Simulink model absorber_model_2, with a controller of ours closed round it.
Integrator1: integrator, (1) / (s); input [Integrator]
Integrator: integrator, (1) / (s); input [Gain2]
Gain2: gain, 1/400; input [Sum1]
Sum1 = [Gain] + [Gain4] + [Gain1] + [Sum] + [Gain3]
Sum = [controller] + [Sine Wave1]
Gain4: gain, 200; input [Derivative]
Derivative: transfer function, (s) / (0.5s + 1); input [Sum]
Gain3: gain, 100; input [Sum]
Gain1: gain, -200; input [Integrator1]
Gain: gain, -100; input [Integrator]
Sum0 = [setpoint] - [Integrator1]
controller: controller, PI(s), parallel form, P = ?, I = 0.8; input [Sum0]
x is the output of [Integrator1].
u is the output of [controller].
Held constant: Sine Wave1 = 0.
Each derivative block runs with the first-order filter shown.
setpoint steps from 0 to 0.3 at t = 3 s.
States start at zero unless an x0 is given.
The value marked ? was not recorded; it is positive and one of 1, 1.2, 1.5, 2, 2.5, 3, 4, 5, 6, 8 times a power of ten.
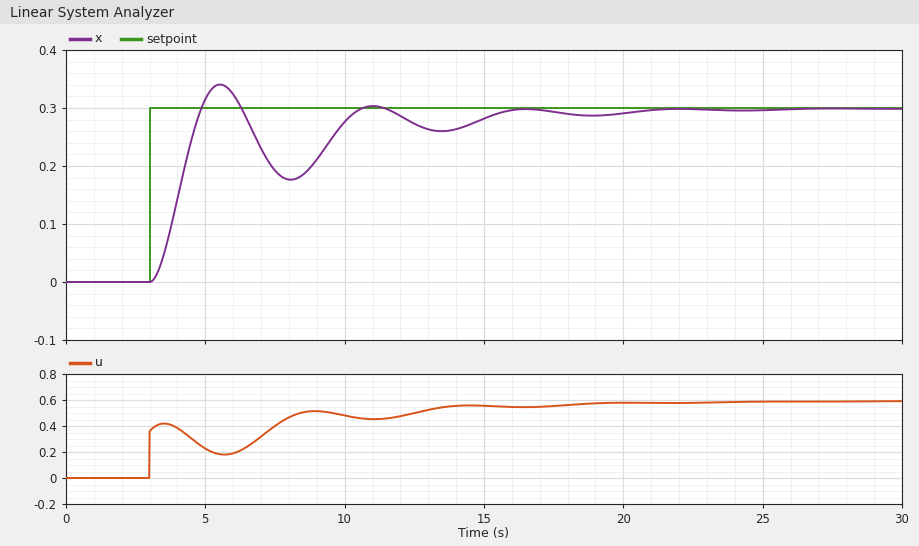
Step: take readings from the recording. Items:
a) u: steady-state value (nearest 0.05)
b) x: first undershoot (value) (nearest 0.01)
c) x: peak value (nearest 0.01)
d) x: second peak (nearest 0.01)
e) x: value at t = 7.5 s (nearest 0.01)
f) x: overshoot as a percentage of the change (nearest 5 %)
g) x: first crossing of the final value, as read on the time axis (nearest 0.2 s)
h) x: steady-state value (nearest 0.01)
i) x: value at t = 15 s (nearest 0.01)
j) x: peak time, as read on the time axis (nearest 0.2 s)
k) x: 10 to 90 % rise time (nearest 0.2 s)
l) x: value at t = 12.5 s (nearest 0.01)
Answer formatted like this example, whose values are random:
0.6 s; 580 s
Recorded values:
0.60; 0.18; 0.34; 0.30; 0.19; 15 %; 4.8 s; 0.30; 0.28; 5.6 s; 1.2 s; 0.27
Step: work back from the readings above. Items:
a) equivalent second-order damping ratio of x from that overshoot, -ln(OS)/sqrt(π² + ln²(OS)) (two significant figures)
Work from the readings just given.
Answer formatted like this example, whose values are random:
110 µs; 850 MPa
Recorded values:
0.52
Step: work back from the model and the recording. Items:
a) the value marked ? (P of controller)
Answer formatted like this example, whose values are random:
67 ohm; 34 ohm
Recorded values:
1.2
